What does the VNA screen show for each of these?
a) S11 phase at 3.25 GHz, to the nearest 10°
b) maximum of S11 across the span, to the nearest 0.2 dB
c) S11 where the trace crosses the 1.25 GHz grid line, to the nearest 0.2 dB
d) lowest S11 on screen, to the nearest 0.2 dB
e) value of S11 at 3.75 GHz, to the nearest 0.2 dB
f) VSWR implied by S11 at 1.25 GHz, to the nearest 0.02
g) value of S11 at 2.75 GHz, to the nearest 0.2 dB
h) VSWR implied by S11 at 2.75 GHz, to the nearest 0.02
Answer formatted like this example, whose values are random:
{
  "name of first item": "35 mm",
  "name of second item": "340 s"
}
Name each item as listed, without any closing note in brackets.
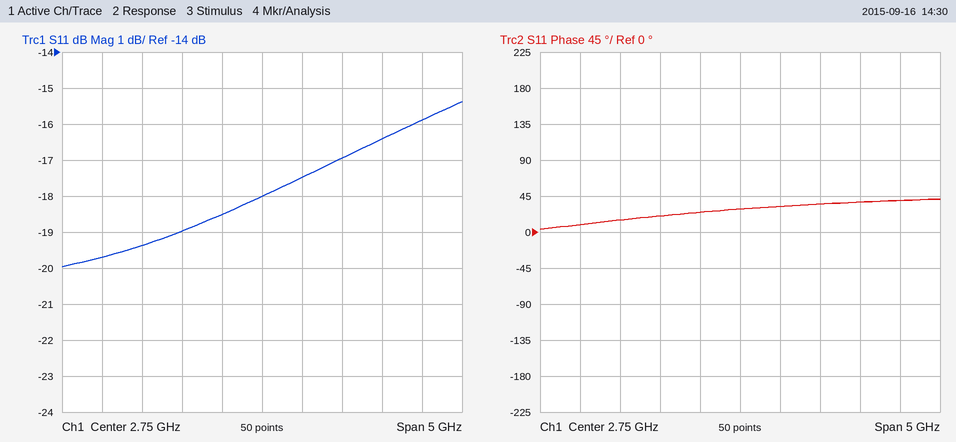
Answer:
{
  "S11 phase at 3.25 GHz, to the nearest 10°": "30°",
  "maximum of S11 across the span, to the nearest 0.2 dB": "-15.4 dB",
  "S11 where the trace crosses the 1.25 GHz grid line, to the nearest 0.2 dB": "-19.4 dB",
  "lowest S11 on screen, to the nearest 0.2 dB": "-20.0 dB",
  "value of S11 at 3.75 GHz, to the nearest 0.2 dB": "-17.0 dB",
  "VSWR implied by S11 at 1.25 GHz, to the nearest 0.02": "1.24",
  "value of S11 at 2.75 GHz, to the nearest 0.2 dB": "-18.0 dB",
  "VSWR implied by S11 at 2.75 GHz, to the nearest 0.02": "1.28"
}
